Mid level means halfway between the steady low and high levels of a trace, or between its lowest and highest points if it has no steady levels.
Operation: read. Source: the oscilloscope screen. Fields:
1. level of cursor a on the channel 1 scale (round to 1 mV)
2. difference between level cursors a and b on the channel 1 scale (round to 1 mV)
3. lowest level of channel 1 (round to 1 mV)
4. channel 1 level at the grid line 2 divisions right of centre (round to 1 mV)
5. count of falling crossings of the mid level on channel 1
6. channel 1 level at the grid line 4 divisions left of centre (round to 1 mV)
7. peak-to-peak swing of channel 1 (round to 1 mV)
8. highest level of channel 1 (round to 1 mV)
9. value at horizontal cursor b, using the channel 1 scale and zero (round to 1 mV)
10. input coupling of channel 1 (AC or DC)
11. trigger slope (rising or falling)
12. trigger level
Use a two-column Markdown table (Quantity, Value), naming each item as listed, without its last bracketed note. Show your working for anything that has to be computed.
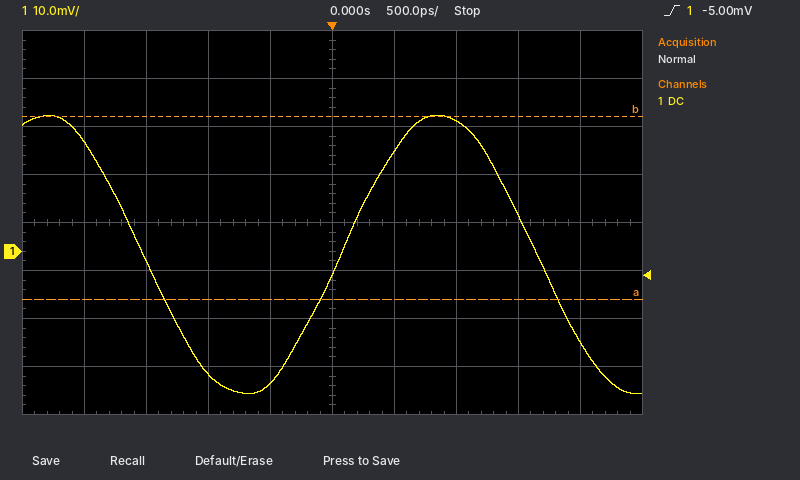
| Quantity | Value |
|---|---|
| level of cursor a on the channel 1 scale | -10 mV |
| difference between level cursors a and b on the channel 1 scale | 38 mV |
| lowest level of channel 1 | -30 mV |
| channel 1 level at the grid line 2 divisions right of centre | 27 mV |
| count of falling crossings of the mid level on channel 1 | 2 |
| channel 1 level at the grid line 4 divisions left of centre | 23 mV |
| peak-to-peak swing of channel 1 | 28 mV − (-30 mV) = 58 mV |
| highest level of channel 1 | 28 mV |
| value at horizontal cursor b, using the channel 1 scale and zero | 28 mV |
| input coupling of channel 1 | DC |
| trigger slope | rising |
| trigger level | -5.00 mV |
